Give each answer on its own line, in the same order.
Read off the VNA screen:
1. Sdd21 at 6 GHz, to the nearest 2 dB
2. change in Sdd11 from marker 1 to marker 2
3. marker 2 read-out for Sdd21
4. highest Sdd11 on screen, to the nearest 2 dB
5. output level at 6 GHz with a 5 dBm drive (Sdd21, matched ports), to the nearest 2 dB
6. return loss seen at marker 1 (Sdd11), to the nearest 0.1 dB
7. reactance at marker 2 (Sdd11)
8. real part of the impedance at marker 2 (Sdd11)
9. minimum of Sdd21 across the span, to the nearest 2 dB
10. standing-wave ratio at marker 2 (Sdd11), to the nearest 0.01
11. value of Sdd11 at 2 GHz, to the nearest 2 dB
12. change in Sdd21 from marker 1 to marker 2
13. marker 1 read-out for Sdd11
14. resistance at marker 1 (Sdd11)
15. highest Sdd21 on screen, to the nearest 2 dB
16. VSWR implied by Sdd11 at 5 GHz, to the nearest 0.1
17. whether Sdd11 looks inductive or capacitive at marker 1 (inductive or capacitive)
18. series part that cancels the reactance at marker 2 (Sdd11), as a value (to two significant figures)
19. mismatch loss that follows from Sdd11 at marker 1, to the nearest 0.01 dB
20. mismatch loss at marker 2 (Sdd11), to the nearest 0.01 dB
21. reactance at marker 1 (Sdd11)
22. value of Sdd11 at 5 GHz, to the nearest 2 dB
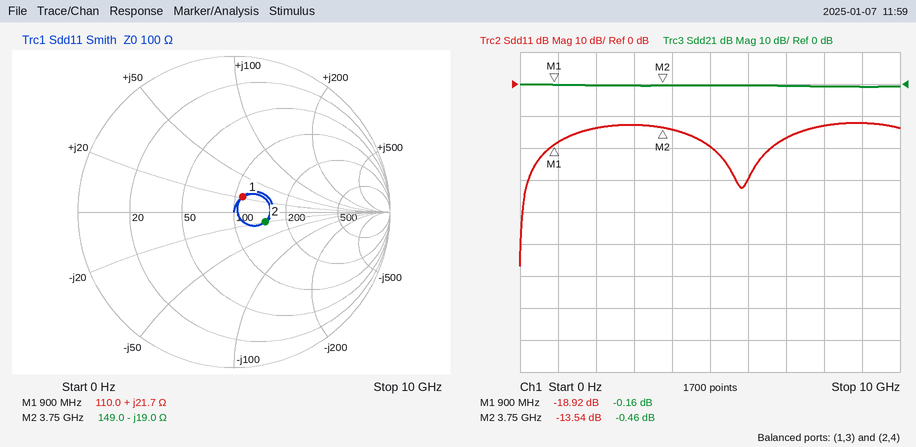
0 dB
5.38 dB
-0.46 dB
-12 dB
4 dBm
18.9 dB
-19.0 Ω
149.0 Ω
0 dB
1.53
-14 dB
-0.30 dB
-18.92 dB
110.0 Ω
0 dB
1.2
inductive
810 pH
0.06 dB
0.20 dB
+21.7 Ω
-20 dB
